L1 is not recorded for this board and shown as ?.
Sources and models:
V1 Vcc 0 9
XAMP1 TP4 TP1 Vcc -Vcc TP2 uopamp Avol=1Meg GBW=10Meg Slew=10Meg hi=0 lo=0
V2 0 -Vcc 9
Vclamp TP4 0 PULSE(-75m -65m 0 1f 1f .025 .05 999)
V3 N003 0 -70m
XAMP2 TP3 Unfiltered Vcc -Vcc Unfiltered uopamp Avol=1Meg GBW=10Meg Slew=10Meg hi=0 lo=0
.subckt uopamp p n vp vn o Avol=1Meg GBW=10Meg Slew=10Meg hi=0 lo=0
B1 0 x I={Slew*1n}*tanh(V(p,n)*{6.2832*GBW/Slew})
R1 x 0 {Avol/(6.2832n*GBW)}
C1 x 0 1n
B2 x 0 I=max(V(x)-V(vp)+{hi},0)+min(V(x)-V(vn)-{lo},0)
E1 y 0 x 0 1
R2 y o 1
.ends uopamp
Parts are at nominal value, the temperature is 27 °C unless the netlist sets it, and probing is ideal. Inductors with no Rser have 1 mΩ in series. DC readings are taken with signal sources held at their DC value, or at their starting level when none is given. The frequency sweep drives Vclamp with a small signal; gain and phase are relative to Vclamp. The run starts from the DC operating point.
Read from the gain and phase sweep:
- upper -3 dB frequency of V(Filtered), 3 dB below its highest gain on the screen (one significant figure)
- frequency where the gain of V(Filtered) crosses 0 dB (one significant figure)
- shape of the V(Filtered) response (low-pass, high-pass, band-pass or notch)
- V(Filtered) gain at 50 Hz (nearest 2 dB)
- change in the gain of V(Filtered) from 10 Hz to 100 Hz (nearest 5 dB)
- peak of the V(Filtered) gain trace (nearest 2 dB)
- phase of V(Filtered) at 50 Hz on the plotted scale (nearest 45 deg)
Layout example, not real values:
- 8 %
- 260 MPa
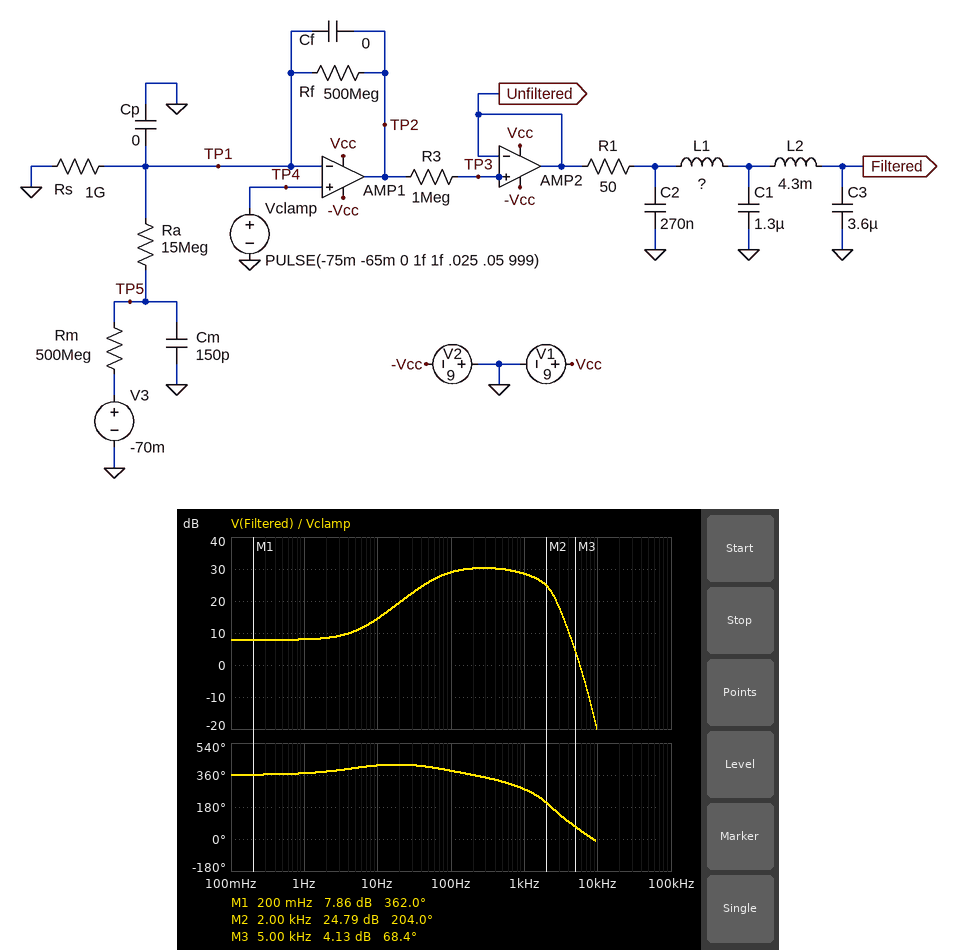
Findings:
- 1 kHz
- 6 kHz
- band-pass
- 26 dB
- 15 dB
- 30 dB
- 405 deg
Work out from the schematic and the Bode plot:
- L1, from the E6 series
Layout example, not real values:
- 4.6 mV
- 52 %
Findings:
- 1.5 mH
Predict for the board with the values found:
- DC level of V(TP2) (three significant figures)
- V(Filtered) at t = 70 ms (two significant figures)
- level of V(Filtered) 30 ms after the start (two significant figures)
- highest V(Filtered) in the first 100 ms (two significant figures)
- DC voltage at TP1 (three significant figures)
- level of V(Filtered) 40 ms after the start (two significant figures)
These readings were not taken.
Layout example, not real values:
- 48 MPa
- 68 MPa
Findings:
- -117 mV
- -93 mV
- -150 mV
- 180 mV
- -75.0 mV
- -120 mV
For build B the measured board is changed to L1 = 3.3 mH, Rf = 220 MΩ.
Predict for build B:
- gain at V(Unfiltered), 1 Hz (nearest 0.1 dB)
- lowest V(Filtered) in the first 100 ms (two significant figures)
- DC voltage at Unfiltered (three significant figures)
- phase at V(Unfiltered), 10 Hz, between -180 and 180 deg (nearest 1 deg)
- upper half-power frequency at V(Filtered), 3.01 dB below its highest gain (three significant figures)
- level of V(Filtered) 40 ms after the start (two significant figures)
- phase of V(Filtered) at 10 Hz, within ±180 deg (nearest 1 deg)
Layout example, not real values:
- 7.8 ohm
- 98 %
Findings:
- 4.4 dB
- -220 mV
- -93.6 mV
- 45 deg
- 1.18 kHz
- -94 mV
- 44 deg
